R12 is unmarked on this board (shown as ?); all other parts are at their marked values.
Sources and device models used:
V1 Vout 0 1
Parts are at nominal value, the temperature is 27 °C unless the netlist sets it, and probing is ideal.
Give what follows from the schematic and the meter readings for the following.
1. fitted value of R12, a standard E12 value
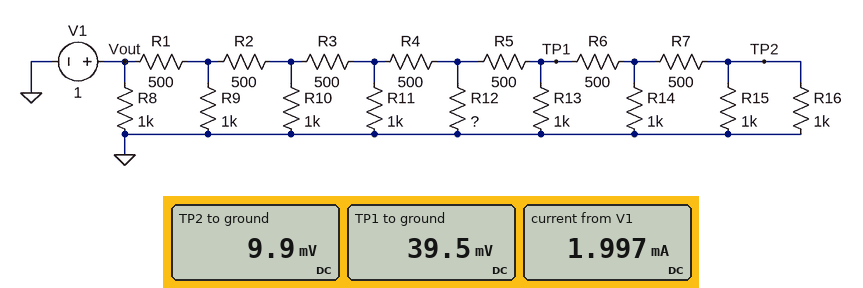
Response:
2.7 kΩ
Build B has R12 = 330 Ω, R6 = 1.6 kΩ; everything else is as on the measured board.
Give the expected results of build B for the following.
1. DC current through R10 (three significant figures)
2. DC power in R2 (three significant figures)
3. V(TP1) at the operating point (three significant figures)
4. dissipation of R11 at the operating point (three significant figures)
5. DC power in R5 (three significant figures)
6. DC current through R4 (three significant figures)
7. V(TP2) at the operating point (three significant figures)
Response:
244 µA
128 µW
22.1 mV
12.8 µW
534 nW
149 µA
2.64 mV
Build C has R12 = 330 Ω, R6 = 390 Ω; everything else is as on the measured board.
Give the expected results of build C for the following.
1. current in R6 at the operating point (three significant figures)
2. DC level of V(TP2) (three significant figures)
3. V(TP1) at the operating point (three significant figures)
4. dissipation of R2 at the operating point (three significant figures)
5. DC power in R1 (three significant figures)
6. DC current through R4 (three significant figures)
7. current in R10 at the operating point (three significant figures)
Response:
20.2 µA
5.06 mV
18.0 mV
129 µW
505 µW
151 µA
244 µA
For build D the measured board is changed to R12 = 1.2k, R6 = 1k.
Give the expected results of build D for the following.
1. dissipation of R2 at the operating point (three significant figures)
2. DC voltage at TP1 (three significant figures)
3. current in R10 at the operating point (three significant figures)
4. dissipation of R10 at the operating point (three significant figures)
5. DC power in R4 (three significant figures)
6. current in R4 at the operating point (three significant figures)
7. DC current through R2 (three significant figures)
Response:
124 µW
37.3 mV
251 µA
63.2 µW
7.09 µW
119 µA
498 µA
